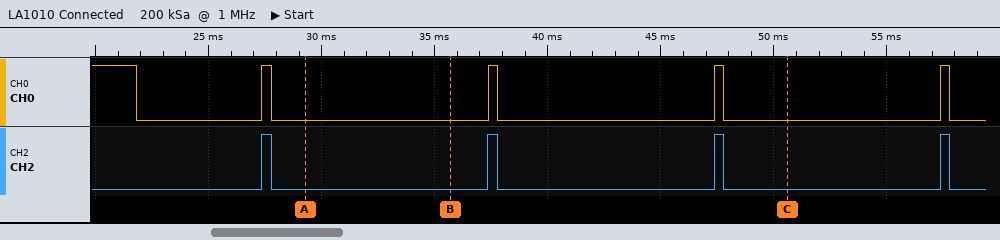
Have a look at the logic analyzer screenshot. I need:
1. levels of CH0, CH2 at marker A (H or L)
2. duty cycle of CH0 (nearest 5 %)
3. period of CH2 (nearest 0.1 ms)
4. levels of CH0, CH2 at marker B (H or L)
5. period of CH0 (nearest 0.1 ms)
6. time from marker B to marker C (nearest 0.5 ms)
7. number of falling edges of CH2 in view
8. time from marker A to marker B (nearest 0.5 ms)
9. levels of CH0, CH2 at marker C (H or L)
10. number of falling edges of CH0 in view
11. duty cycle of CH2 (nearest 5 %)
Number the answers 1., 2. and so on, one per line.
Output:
1. CH0=L, CH2=L
2. 5 %
3. 10 ms
4. CH0=L, CH2=L
5. 10 ms
6. 15 ms
7. 4
8. 6.5 ms
9. CH0=L, CH2=L
10. 5
11. 5 %
